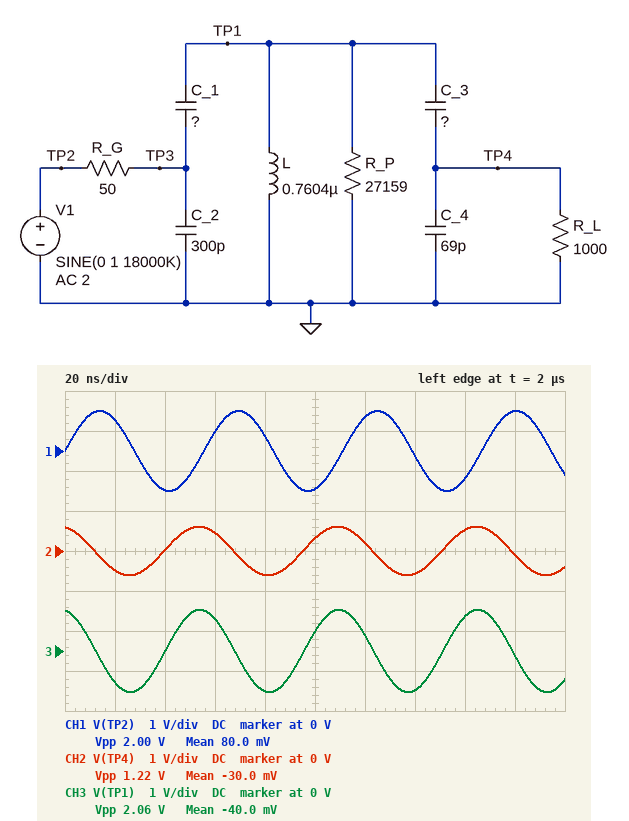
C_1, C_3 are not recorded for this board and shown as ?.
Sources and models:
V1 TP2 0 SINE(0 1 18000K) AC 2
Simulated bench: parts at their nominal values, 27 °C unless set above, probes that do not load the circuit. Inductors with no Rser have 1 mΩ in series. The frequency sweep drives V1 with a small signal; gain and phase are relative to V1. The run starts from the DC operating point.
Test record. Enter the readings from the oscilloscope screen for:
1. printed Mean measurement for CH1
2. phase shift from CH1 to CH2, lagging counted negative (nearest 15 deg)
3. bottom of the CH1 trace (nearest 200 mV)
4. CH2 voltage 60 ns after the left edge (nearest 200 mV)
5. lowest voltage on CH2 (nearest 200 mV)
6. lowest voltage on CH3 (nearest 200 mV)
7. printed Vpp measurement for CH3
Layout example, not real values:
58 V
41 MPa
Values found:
80.0 mV
105 deg
-1.0 V
400 mV
-600 mV
-1.0 V
2.06 V
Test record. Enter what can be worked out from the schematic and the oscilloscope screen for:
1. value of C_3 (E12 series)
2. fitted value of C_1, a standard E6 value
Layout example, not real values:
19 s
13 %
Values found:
100 pF
47 pF
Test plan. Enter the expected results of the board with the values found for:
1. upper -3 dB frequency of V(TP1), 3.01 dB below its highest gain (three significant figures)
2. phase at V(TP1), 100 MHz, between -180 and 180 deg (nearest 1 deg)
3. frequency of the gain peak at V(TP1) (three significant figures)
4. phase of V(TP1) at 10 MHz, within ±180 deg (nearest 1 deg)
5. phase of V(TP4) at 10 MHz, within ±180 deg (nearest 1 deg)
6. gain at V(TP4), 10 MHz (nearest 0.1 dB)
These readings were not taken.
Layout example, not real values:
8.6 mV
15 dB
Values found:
20.8 MHz
-84 deg
20.1 MHz
130 deg
136 deg
-22.5 dB
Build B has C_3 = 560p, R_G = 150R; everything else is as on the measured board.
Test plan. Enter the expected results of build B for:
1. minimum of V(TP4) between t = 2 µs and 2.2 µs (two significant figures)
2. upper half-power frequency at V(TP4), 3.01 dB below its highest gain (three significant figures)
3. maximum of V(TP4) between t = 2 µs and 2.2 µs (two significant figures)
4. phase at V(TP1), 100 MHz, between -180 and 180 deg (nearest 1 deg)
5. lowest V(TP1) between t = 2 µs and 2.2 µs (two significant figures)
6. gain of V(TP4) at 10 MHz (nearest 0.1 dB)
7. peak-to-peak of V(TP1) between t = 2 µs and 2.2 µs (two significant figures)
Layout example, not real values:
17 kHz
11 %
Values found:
-830 mV
18.8 MHz
830 mV
-87 deg
-940 mV
-25.5 dB
1.9 V
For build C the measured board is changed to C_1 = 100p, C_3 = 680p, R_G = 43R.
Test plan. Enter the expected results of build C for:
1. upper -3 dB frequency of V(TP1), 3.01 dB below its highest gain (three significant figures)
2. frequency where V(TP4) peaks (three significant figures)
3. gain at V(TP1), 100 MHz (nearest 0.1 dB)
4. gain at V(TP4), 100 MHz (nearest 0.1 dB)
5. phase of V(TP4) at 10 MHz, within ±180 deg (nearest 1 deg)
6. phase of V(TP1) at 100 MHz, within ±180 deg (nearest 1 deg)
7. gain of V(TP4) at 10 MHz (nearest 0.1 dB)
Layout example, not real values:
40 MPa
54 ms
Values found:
16.3 MHz
15.2 MHz
-23.3 dB
-24.1 dB
126 deg
-83 deg
-9.6 dB
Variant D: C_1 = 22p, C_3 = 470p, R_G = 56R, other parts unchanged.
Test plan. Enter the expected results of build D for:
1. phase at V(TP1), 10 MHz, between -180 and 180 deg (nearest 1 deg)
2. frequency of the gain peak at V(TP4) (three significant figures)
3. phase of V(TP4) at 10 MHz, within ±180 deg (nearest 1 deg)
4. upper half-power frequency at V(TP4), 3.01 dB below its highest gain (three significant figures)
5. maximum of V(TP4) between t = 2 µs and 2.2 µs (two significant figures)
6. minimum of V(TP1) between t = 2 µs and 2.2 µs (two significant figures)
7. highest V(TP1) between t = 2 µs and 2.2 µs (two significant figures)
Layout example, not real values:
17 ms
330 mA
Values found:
128 deg
20.3 MHz
130 deg
21.2 MHz
370 mV
-420 mV
420 mV
